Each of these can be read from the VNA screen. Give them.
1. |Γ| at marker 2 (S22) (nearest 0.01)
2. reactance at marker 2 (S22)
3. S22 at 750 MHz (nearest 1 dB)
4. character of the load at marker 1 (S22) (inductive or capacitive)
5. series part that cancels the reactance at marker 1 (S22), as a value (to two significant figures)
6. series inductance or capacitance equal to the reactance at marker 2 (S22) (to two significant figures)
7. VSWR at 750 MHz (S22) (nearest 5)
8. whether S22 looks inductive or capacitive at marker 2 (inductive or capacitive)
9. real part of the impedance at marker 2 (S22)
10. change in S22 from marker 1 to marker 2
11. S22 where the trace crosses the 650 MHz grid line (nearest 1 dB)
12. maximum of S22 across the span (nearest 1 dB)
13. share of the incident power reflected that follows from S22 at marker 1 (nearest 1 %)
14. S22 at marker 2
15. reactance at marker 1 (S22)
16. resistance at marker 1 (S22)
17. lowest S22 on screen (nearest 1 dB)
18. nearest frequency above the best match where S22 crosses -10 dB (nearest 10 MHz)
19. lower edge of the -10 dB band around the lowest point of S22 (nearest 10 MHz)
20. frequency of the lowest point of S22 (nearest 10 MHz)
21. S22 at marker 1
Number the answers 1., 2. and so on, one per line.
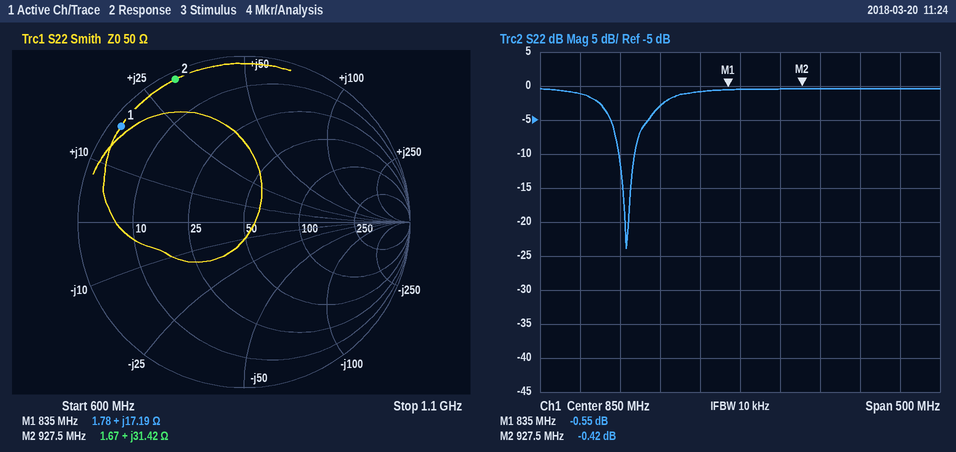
1. 0.95
2. +31.42 Ω
3. -3 dB
4. inductive
5. 11 pF
6. 5.4 nH
7. 5
8. inductive
9. 1.67 Ω
10. 0.13 dB
11. -1 dB
12. 0 dB
13. 88 %
14. -0.42 dB
15. +17.19 Ω
16. 1.78 Ω
17. -24 dB
18. 720 MHz
19. 700 MHz
20. 710 MHz
21. -0.55 dB
